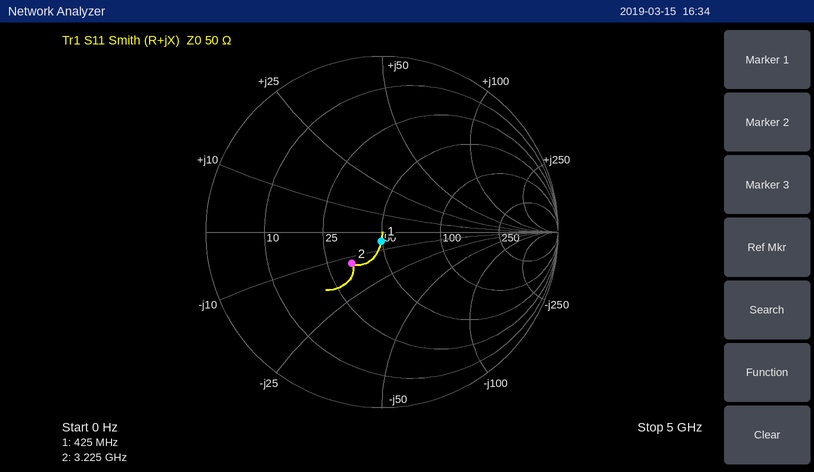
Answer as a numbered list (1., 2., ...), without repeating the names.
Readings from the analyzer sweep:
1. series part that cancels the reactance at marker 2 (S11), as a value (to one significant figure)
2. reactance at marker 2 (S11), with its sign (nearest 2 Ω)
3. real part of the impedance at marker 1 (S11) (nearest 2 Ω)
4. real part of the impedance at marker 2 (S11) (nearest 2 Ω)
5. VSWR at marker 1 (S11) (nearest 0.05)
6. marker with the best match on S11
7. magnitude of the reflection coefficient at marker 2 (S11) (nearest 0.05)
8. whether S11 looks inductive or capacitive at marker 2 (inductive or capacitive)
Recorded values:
1. 600 pH
2. -12 Ω
3. 50 Ω
4. 34 Ω
5. 1.10
6. marker 1
7. 0.25
8. capacitive
